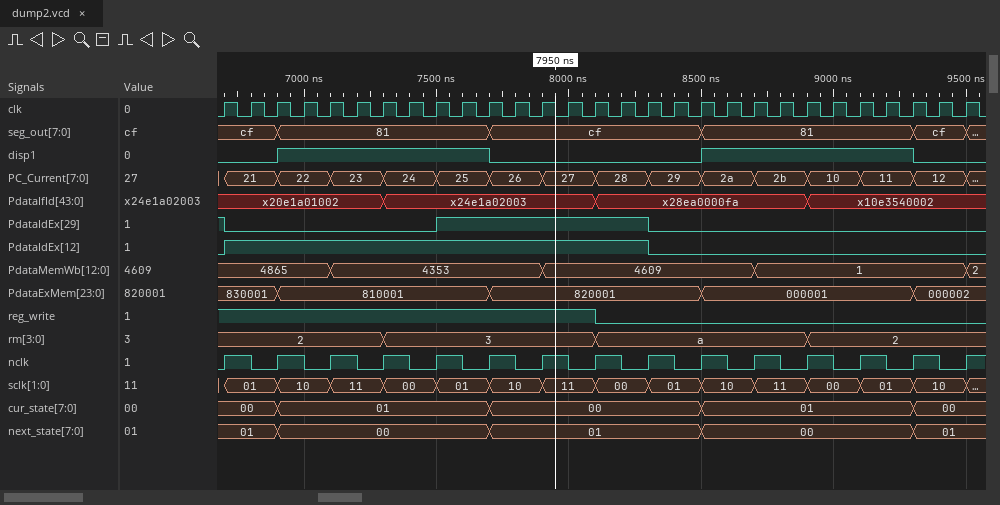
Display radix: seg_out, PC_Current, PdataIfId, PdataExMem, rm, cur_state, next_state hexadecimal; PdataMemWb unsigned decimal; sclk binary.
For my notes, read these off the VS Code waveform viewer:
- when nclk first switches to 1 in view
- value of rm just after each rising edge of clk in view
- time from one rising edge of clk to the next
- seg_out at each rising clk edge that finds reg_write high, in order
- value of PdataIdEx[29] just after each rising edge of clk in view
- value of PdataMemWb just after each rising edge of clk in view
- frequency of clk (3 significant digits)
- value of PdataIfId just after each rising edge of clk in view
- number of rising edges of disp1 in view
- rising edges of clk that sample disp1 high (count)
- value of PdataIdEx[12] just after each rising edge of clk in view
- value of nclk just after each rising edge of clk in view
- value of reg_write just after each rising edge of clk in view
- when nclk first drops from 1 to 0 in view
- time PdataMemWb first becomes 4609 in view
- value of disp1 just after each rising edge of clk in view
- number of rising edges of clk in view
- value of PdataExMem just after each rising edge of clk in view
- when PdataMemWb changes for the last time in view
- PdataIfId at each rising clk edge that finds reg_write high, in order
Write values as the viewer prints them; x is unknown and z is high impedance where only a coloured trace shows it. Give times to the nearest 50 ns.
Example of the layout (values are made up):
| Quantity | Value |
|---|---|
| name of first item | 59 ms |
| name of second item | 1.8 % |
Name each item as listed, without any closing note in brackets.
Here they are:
| Quantity | Value |
|---|---|
| when nclk first switches to 1 in view | 6700 ns |
| value of rm just after each rising edge of clk in view | 2, 2, 2, 2, 2, 2, 3, 3, 3, 3, 3, 3, 3, 3, a, a, a, a, a, a, a, a, 2, 2, 2, 2, 2, 2, 2 |
| time from one rising edge of clk to the next | 100 ns |
| seg_out at each rising clk edge that finds reg_write high, in order | cf, cf, cf, 81, 81, 81, 81, 81, 81, 81, 81, cf, cf, cf, cf |
| value of PdataIdEx[29] just after each rising edge of clk in view | 0 0 0 0 0 0 0 0 1 1 1 1 1 1 1 1 0 0 0 0 0 0 0 0 0 0 0 0 0 |
| value of PdataMemWb just after each rising edge of clk in view | 4865, 4865, 4865, 4865, 4353, 4353, 4353, 4353, 4353, 4353, 4353, 4353, 4609, 4609, 4609, 4609, 4609, 4609, 4609, 4609, 1, 1, 1, 1, 1, 1, 1, 1, 2 |
| frequency of clk | 10.0 MHz |
| value of PdataIfId just after each rising edge of clk in view | x20e1a01002, x20e1a01002, x20e1a01002, x20e1a01002, x20e1a01002, x20e1a01002, x24e1a02003, x24e1a02003, x24e1a02003, x24e1a02003, x24e1a02003, x24e1a02003, x24e1a02003, x24e1a02003, x28ea0000fa, x28ea0000fa, x28ea0000fa, x28ea0000fa, x28ea0000fa, x28ea0000fa, x28ea0000fa, x28ea0000fa, x10e3540002, x10e3540002, x10e3540002, x10e3540002, x10e3540002, x10e3540002, x10e3540002 |
| number of rising edges of disp1 in view | 2 |
| rising edges of clk that sample disp1 high | 16 |
| value of PdataIdEx[12] just after each rising edge of clk in view | 1 1 1 1 1 1 1 1 1 1 1 1 1 1 1 1 0 0 0 0 0 0 0 0 0 0 0 0 0 |
| value of nclk just after each rising edge of clk in view | 1 0 1 0 1 0 1 0 1 0 1 0 1 0 1 0 1 0 1 0 1 0 1 0 1 0 1 0 1 |
| value of reg_write just after each rising edge of clk in view | 1 1 1 1 1 1 1 1 1 1 1 1 1 1 0 0 0 0 0 0 0 0 0 0 0 0 0 0 0 |
| when nclk first drops from 1 to 0 in view | 6800 ns |
| time PdataMemWb first becomes 4609 in view | 7900 ns |
| value of disp1 just after each rising edge of clk in view | 0 0 1 1 1 1 1 1 1 1 0 0 0 0 0 0 0 0 1 1 1 1 1 1 1 1 0 0 0 |
| number of rising edges of clk in view | 29 |
| value of PdataExMem just after each rising edge of clk in view | 830001, 830001, 810001, 810001, 810001, 810001, 810001, 810001, 810001, 810001, 820001, 820001, 820001, 820001, 820001, 820001, 820001, 820001, 000001, 000001, 000001, 000001, 000001, 000001, 000001, 000001, 000002, 000002, 000002 |
| when PdataMemWb changes for the last time in view | 9500 ns |
| PdataIfId at each rising clk edge that finds reg_write high, in order | x20e1a01002, x20e1a01002, x20e1a01002, x20e1a01002, x20e1a01002, x20e1a01002, x20e1a01002, x24e1a02003, x24e1a02003, x24e1a02003, x24e1a02003, x24e1a02003, x24e1a02003, x24e1a02003, x24e1a02003 |
